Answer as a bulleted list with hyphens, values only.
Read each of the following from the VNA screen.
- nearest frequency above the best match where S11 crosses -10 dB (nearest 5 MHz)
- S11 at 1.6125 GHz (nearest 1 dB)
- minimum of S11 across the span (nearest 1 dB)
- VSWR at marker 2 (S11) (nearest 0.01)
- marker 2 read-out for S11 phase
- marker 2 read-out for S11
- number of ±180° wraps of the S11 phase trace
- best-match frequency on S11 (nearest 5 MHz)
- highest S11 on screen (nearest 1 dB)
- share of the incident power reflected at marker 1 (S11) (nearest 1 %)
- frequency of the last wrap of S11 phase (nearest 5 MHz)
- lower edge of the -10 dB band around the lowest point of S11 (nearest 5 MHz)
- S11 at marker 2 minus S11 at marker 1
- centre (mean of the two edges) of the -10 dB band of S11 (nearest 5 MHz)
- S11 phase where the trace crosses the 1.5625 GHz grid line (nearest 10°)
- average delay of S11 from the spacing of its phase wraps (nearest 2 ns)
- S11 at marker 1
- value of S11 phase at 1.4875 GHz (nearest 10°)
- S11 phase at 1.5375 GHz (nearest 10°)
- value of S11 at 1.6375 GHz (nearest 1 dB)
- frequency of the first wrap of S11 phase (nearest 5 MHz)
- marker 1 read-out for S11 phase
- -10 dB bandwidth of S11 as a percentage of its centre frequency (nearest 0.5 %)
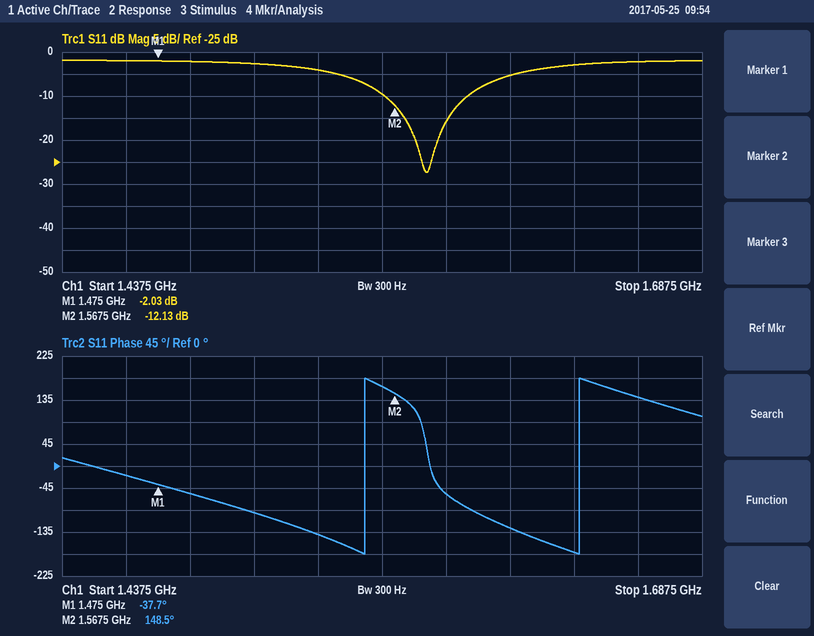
- 1.595 GHz
- -5 dB
- -27 dB
- 1.66
- 148.5°
- -12.13 dB
- 2
- 1.580 GHz
- -2 dB
- 63 %
- 1.640 GHz
- 1.565 GHz
- -10.10 dB
- 1.580 GHz
- 160°
- 12 ns
- -2.03 dB
- -60°
- -140°
- -3 dB
- 1.555 GHz
- -37.7°
- 2.0 %
